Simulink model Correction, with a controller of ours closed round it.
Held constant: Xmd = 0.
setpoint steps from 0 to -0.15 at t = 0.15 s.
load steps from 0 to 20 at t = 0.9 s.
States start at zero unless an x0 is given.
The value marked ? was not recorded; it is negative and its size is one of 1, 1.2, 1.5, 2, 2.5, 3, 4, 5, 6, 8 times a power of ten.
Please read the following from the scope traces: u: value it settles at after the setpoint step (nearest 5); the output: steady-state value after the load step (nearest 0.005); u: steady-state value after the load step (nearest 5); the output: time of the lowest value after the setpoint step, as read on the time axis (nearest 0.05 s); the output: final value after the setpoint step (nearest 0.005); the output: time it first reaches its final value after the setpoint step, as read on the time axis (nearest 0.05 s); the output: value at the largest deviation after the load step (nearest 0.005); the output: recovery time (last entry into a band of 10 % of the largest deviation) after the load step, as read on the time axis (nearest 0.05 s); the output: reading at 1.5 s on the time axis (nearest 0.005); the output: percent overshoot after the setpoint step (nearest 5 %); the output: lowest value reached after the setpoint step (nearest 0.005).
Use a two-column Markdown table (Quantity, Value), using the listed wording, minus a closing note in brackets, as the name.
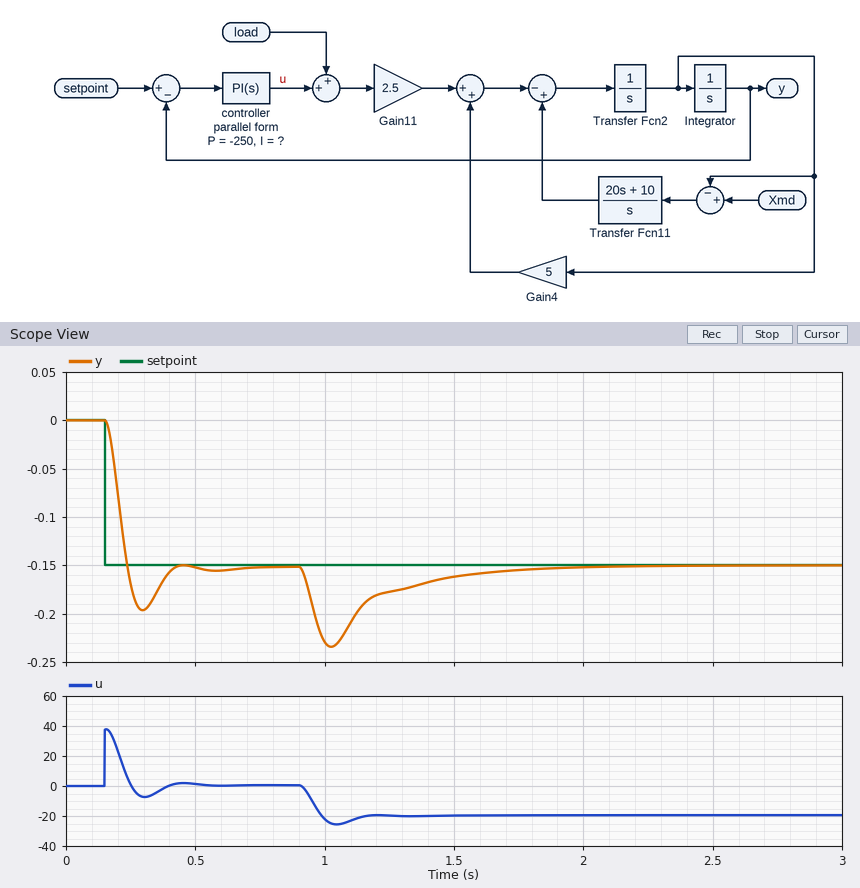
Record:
| Quantity | Value |
|---|---|
| u: value it settles at after the setpoint step | 0 |
| the output: steady-state value after the load step | -0.150 |
| u: steady-state value after the load step | -20 |
| the output: time of the lowest value after the setpoint step, as read on the time axis | 0.30 s |
| the output: final value after the setpoint step | -0.150 |
| the output: time it first reaches its final value after the setpoint step, as read on the time axis | 0.25 s |
| the output: value at the largest deviation after the load step | -0.235 |
| the output: recovery time (last entry into a band of 10 % of the largest deviation) after the load step, as read on the time axis | 1.60 s |
| the output: reading at 1.5 s on the time axis | -0.160 |
| the output: percent overshoot after the setpoint step | 30 % |
| the output: lowest value reached after the setpoint step | -0.195 |
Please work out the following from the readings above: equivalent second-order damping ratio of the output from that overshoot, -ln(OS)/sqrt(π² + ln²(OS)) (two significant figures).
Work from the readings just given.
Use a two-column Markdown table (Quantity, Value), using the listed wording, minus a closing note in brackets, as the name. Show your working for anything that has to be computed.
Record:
| Quantity | Value |
|---|---|
| equivalent second-order damping ratio of the output from that overshoot, -ln(OS)/sqrt(π² + ln²(OS)) | ln(0.3) = -1.204; 1.204 / sqrt(9.870 + 1.450) = 0.36 |
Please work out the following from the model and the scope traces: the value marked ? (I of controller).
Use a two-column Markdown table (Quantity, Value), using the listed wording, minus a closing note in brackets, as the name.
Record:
| Quantity | Value |
|---|---|
| the value marked ? | -800 |
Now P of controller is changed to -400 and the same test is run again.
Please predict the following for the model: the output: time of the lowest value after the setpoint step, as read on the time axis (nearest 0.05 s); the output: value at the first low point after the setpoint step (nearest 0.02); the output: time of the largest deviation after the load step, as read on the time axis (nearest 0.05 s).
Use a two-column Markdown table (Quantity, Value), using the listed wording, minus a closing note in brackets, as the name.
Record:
| Quantity | Value |
|---|---|
| the output: time of the lowest value after the setpoint step, as read on the time axis | 0.25 s |
| the output: value at the first low point after the setpoint step | -0.20 |
| the output: time of the largest deviation after the load step, as read on the time axis | 1.00 s |
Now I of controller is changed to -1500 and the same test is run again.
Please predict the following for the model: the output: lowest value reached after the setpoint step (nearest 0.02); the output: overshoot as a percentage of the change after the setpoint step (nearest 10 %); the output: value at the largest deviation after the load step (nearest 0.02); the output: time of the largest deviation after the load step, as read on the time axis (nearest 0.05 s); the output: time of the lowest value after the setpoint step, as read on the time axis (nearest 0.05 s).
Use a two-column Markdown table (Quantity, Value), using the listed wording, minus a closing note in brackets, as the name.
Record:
| Quantity | Value |
|---|---|
| the output: lowest value reached after the setpoint step | -0.22 |
| the output: overshoot as a percentage of the change after the setpoint step | 40 % |
| the output: value at the largest deviation after the load step | -0.22 |
| the output: time of the largest deviation after the load step, as read on the time axis | 1.00 s |
| the output: time of the lowest value after the setpoint step, as read on the time axis | 0.30 s |
